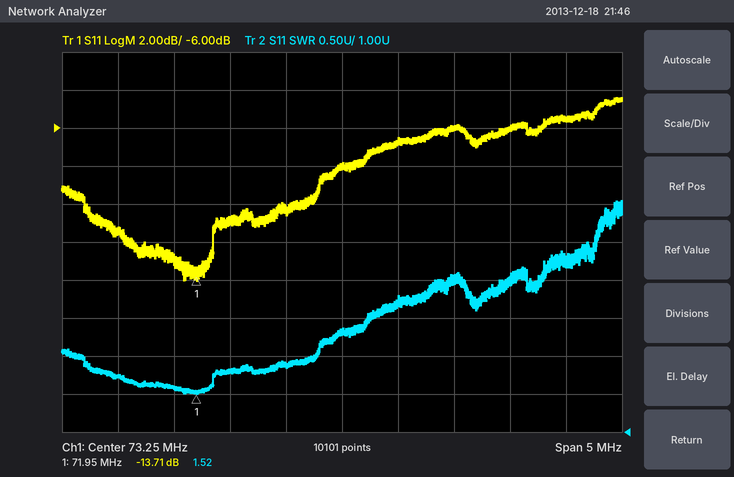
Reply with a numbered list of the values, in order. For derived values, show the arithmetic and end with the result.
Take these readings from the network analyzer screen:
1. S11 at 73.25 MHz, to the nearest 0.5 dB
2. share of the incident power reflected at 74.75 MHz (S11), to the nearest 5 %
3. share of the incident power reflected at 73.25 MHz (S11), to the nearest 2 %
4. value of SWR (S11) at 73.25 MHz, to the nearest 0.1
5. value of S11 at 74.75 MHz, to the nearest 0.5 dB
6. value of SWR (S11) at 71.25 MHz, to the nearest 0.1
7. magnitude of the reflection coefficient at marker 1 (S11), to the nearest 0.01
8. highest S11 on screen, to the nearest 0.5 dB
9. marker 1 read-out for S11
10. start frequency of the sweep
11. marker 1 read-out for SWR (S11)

1. -8.0 dB
2. 10^(-6/10) ≈ 25 %
3. 10^(-8/10) ≈ 16 %
4. 2.3
5. -6.0 dB
6. 1.7
7. 10^(-13.71/20) ≈ 0.21
8. -4.5 dB
9. -13.71 dB
10. 70.75 MHz
11. 1.52
